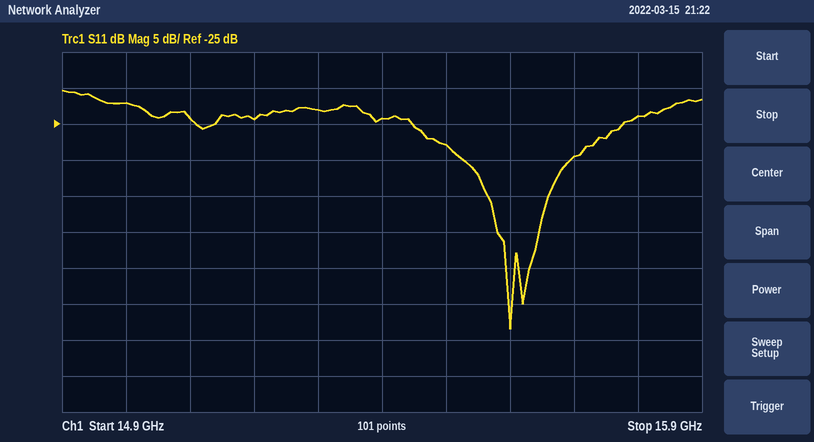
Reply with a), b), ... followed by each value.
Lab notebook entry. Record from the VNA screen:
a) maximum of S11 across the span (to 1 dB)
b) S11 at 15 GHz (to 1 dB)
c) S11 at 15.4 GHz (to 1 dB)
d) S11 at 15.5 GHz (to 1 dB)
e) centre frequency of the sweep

a) -20 dB
b) -22 dB
c) -24 dB
d) -28 dB
e) 15.4 GHz
